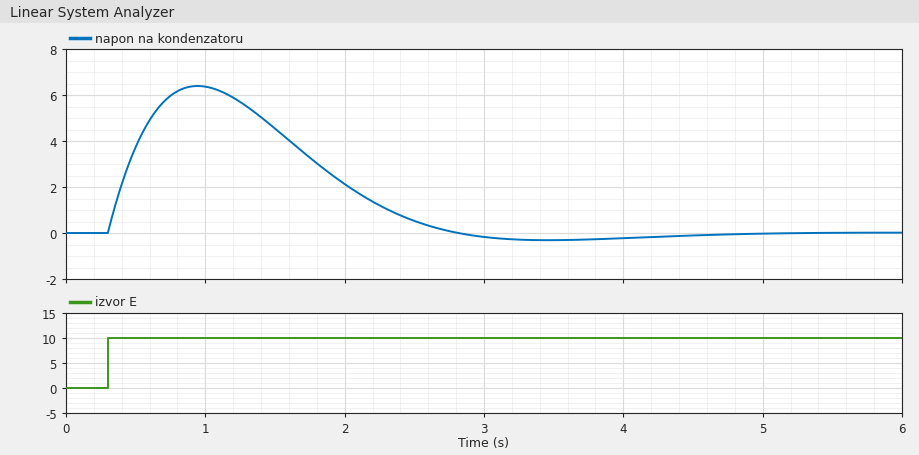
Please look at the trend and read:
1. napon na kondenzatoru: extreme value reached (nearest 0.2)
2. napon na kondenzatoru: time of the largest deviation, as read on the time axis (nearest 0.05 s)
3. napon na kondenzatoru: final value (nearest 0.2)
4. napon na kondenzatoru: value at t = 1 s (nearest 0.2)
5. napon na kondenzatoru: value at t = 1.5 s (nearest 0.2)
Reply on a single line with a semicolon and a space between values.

6.4; 0.95 s; 0.0; 6.4; 4.6
